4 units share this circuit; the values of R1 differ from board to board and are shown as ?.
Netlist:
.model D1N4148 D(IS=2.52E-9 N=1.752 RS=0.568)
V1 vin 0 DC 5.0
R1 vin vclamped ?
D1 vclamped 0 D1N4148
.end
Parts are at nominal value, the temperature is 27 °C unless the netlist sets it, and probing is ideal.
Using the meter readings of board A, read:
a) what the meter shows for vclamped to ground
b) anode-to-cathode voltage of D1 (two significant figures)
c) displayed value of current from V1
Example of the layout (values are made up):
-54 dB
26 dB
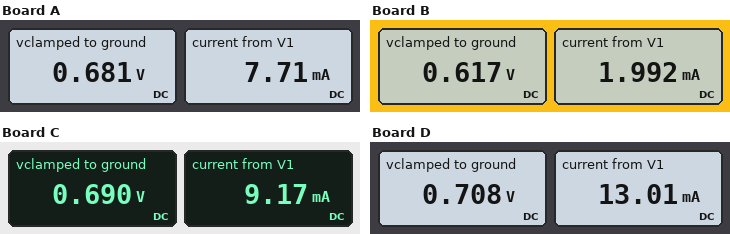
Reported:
0.681 V
680 mV
7.71 mA
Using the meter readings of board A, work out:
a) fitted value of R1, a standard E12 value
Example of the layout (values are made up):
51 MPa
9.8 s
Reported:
560 Ω
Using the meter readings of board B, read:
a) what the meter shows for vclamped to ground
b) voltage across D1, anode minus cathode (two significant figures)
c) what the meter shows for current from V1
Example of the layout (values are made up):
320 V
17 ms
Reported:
0.617 V
620 mV
1.992 mA
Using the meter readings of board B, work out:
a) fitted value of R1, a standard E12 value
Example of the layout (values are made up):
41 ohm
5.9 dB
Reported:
2.2 kΩ
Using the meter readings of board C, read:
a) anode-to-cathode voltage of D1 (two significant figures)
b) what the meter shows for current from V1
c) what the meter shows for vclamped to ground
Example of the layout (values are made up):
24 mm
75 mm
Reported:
690 mV
9.17 mA
0.690 V
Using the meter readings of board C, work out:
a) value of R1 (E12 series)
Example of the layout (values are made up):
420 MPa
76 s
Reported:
470 Ω
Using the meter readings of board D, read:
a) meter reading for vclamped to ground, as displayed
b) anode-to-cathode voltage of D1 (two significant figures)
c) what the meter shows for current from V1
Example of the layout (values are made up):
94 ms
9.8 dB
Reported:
0.708 V
710 mV
13.01 mA
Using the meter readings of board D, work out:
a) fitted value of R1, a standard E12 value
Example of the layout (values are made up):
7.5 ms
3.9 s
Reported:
330 Ω
